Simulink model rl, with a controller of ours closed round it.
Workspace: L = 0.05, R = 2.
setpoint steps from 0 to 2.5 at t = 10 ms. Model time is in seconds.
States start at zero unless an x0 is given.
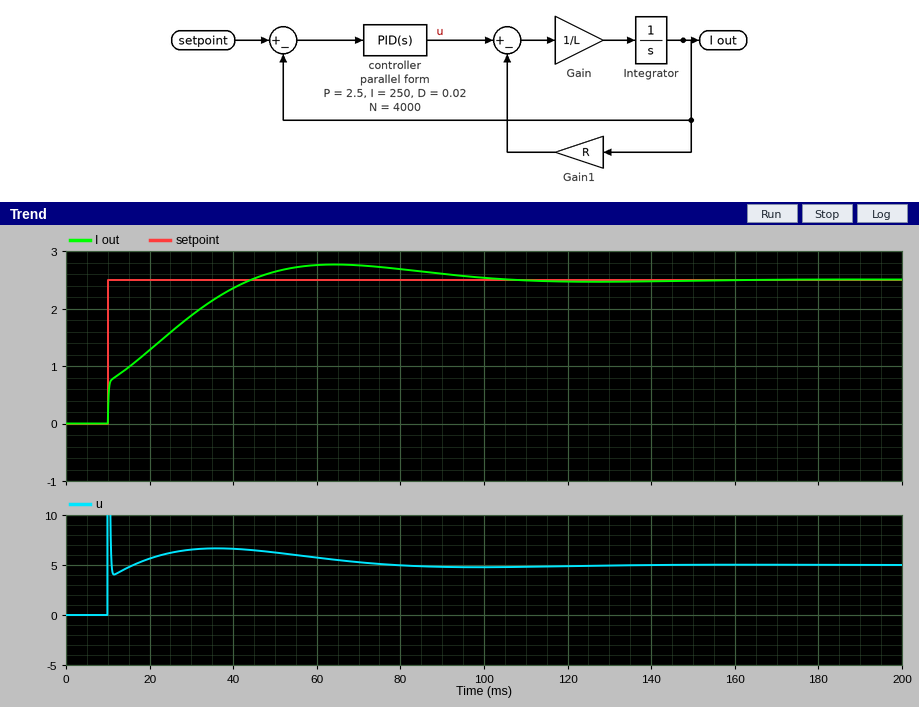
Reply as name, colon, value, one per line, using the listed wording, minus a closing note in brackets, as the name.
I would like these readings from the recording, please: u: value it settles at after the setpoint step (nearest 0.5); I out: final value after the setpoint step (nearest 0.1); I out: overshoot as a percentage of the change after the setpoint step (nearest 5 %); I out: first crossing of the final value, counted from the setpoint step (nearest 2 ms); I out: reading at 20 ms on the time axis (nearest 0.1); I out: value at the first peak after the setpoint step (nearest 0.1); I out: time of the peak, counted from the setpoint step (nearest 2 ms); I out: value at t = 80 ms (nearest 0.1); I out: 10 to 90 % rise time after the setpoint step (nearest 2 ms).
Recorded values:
u: value it settles at after the setpoint step: 5.0
I out: final value after the setpoint step: 2.5
I out: overshoot as a percentage of the change after the setpoint step: 10 %
I out: first crossing of the final value, counted from the setpoint step: 34 ms
I out: reading at 20 ms on the time axis: 1.3
I out: value at the first peak after the setpoint step: 2.8
I out: time of the peak, counted from the setpoint step: 54 ms
I out: value at t = 80 ms: 2.7
I out: 10 to 90 % rise time after the setpoint step: 28 ms
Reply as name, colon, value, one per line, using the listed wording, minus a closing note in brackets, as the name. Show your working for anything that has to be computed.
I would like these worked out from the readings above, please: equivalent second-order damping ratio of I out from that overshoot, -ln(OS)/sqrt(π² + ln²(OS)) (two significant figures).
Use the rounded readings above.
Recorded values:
equivalent second-order damping ratio of I out from that overshoot, -ln(OS)/sqrt(π² + ln²(OS)): ln(0.1) = -2.303; 2.303 / sqrt(9.870 + 5.302) = 0.59
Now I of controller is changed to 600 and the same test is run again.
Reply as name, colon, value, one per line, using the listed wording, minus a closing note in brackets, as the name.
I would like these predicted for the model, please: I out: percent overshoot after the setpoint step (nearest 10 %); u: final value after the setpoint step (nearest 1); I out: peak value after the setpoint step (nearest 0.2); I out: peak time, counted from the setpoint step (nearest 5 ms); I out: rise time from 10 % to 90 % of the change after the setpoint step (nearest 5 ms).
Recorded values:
I out: percent overshoot after the setpoint step: 20 %
u: final value after the setpoint step: 5
I out: peak value after the setpoint step: 3.0
I out: peak time, counted from the setpoint step: 35 ms
I out: rise time from 10 % to 90 % of the change after the setpoint step: 15 ms
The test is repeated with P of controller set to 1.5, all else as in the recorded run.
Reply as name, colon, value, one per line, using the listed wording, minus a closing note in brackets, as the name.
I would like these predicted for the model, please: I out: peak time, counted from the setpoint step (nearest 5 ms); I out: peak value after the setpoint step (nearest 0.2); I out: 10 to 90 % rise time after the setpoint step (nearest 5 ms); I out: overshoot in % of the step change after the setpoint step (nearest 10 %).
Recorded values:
I out: peak time, counted from the setpoint step: 55 ms
I out: peak value after the setpoint step: 3.0
I out: 10 to 90 % rise time after the setpoint step: 30 ms
I out: overshoot in % of the step change after the setpoint step: 20 %
